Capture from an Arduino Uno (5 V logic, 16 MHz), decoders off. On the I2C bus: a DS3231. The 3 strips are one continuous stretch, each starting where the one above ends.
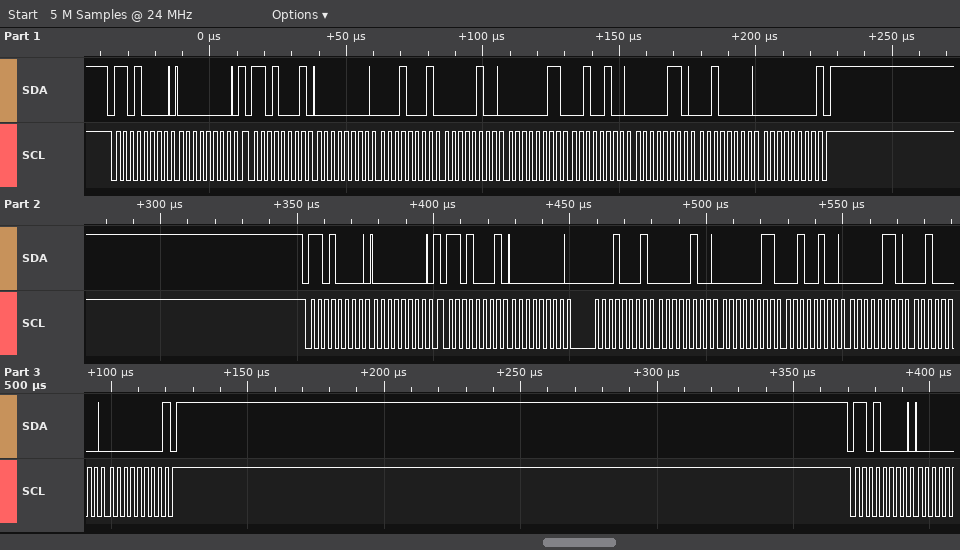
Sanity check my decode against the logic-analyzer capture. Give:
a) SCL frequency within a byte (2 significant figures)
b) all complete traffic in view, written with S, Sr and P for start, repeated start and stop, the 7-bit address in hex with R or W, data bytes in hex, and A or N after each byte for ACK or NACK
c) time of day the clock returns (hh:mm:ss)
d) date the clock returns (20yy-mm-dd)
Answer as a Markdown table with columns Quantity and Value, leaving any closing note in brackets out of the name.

| Quantity | Value |
|---|---|
| SCL frequency within a byte | 400 kHz |
| all complete traffic in view, written with S, Sr and P for start, repeated start and stop, the 7-bit address in hex with R or W, data bytes in hex, and A or N after each byte for ACK or NACK | S 68W A 00 A Sr 68R A 00 A 11 A 04 A 03 A 24 A 06 A 20 A 00 N P S 68W A 00 A Sr 68R A 00 A 11 A 04 A 03 A 24 A 06 A 20 A 00 N P S 68W A |
| time of day the clock returns | 04:11:00 |
| date the clock returns | 2020-06-24 |
